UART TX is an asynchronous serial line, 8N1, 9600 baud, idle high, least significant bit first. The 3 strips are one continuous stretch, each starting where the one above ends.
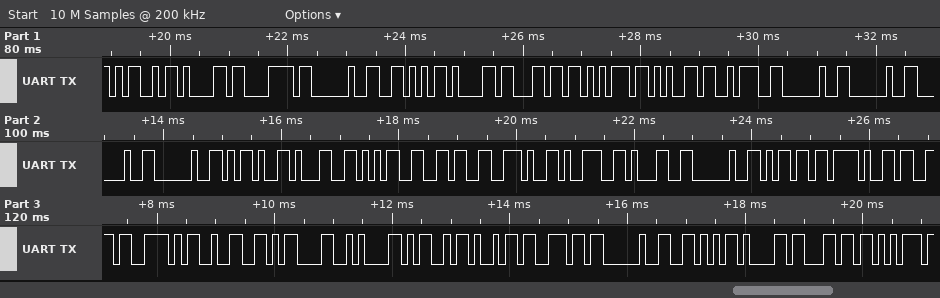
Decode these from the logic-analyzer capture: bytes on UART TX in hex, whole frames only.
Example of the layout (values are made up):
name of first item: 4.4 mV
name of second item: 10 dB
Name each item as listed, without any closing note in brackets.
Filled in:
bytes on UART TX in hex, whole frames only: 4D 61 78 20 56 61 6C 75 65 3A 20 20 20 20 2D 31 35 36 2E 39 31 20 6D 2F 73 5E 32 0D 0A 4D 69 6E 20 56 61 6C 75
